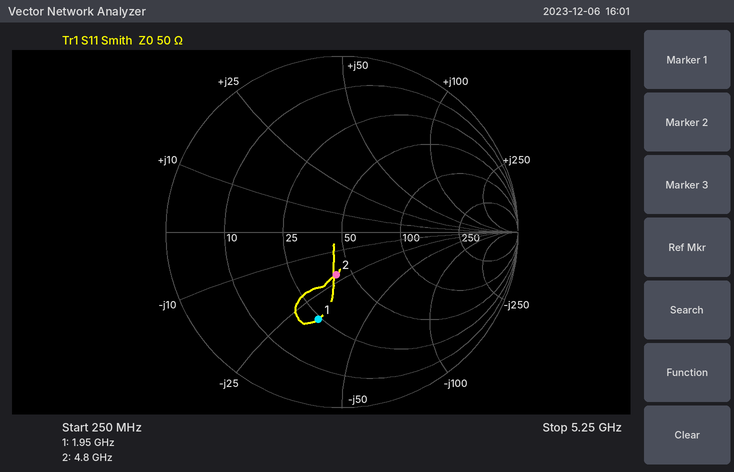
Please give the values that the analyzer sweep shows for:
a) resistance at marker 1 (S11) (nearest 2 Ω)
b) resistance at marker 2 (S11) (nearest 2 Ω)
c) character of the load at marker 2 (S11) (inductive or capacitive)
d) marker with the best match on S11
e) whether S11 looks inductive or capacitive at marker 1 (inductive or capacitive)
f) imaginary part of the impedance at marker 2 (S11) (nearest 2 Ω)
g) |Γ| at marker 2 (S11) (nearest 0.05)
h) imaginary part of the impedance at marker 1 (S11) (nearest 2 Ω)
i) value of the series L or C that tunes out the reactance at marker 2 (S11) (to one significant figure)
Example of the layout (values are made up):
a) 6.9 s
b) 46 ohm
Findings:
a) 24 Ω
b) 42 Ω
c) capacitive
d) marker 2
e) capacitive
f) -22 Ω
g) 0.25
h) -32 Ω
i) 700 pH
